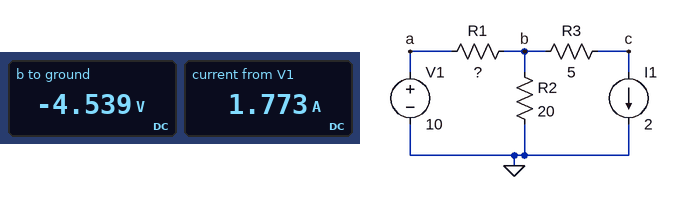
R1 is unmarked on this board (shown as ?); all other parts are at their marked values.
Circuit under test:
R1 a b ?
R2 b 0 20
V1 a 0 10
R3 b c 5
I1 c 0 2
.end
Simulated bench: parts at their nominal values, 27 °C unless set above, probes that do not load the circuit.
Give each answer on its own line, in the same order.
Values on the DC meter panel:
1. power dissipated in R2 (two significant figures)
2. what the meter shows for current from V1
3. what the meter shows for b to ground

1.0 W
1.773 A
-4.539 V
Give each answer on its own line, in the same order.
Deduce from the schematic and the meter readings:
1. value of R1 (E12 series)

8.2 Ω
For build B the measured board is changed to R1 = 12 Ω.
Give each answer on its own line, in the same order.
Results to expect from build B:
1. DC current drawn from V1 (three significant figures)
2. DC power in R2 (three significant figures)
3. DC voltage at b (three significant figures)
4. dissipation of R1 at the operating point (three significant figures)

1.56 A
3.83 W
-8.75 V
29.3 W
